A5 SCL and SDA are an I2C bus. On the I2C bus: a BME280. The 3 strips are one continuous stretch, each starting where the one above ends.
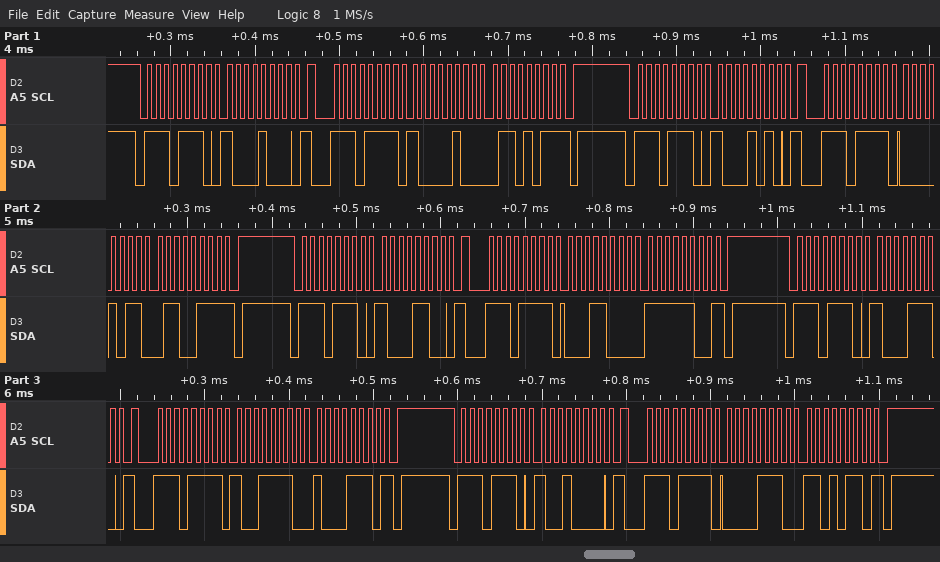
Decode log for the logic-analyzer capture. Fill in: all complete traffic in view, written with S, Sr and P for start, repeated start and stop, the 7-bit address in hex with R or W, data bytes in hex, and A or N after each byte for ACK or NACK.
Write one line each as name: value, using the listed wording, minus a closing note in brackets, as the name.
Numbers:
all complete traffic in view, written with S, Sr and P for start, repeated start and stop, the 7-bit address in hex with R or W, data bytes in hex, and A or N after each byte for ACK or NACK: S 77W A 88 A Sr 77R A 84 A 6B N P S 77W A 8A A Sr 77R A 0B A 67 N P S 77W A 8C A Sr 77R A 18 A FC N P S 77W A 8E A Sr 77R A 9E A 8E N P S 77W A 90 A Sr 77R A 0E A D6 N P
